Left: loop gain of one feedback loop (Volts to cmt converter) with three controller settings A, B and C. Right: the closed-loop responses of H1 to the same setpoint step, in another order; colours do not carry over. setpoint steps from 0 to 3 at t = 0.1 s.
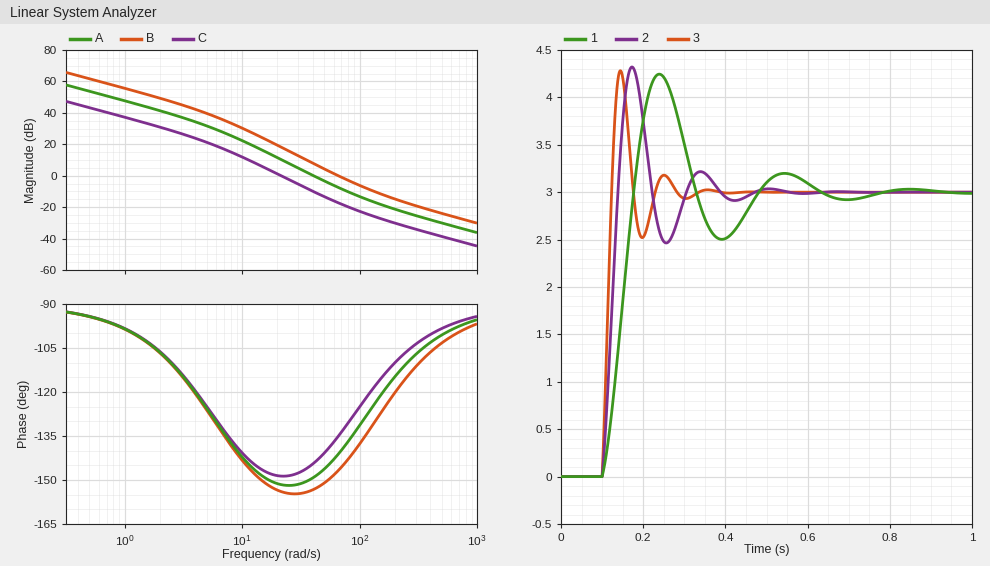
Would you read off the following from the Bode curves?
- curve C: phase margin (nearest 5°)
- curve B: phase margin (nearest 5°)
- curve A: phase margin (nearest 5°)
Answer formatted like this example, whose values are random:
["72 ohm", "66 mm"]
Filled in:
["30°", "35°", "30°"]
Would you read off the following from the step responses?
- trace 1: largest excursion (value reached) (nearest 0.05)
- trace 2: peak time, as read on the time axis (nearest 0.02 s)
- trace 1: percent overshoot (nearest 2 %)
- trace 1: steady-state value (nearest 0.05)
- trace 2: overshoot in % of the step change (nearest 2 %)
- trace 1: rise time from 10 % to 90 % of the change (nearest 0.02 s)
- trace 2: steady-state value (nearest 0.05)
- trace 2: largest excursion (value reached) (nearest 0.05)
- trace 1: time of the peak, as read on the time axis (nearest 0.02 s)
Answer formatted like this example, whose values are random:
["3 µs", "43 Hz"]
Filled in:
["4.25", "0.18 s", "42 %", "3.00", "44 %", "0.06 s", "3.00", "4.30", "0.24 s"]
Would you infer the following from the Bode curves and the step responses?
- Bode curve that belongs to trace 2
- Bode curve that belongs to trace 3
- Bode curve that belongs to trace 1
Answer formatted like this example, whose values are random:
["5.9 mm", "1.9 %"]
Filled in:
["A", "B", "C"]
